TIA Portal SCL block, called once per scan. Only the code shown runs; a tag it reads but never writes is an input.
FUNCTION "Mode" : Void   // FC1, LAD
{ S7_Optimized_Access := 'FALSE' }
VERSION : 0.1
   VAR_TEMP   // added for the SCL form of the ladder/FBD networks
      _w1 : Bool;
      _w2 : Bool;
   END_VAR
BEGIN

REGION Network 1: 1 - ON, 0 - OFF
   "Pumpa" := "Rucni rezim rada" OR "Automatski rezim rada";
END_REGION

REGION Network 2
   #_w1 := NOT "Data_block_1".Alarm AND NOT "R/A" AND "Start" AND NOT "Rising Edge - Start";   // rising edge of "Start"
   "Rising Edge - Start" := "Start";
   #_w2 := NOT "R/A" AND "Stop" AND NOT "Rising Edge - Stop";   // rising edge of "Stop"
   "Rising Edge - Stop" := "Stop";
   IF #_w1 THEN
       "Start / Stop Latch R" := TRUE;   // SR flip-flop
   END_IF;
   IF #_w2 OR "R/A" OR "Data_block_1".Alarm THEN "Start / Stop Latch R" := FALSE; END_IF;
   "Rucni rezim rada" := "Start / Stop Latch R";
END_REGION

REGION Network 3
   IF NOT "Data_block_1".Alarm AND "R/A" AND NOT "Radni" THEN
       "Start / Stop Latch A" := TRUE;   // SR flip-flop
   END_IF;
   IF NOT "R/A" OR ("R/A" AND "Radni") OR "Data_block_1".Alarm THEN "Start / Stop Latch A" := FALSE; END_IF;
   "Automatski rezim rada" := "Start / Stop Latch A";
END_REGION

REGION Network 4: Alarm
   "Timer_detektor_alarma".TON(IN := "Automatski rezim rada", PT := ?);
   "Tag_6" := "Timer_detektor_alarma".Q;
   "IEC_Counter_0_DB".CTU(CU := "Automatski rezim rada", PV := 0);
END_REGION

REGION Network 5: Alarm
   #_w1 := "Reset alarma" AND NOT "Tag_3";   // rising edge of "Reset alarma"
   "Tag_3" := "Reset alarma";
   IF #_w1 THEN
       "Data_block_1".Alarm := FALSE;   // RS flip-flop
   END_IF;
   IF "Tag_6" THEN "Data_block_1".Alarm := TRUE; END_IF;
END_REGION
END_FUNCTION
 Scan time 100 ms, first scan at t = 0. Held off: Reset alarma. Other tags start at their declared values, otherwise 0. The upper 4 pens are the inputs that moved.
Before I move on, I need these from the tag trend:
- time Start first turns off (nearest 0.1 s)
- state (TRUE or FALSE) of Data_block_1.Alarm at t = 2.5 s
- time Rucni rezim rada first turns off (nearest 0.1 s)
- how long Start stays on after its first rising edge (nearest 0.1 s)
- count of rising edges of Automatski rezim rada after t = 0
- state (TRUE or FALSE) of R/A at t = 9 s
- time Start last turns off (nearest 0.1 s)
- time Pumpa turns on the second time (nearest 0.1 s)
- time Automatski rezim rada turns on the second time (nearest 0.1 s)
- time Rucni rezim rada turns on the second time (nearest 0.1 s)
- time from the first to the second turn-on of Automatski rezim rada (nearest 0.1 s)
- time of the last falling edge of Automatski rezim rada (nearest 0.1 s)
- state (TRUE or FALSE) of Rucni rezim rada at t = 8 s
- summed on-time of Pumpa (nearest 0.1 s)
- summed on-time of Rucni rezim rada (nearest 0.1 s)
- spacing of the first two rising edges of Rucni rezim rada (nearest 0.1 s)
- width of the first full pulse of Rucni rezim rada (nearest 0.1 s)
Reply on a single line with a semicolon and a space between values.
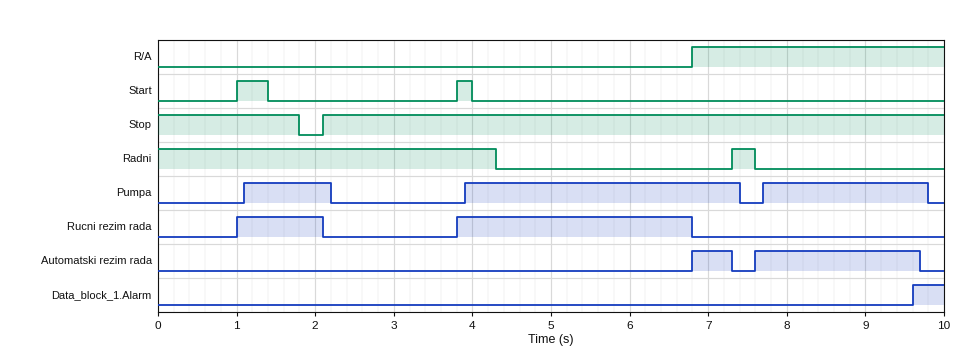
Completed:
1.4 s; FALSE; 2.1 s; 0.4 s; 2; TRUE; 4.0 s; 3.9 s; 7.6 s; 3.8 s; 0.8 s; 9.7 s; FALSE; 6.7 s; 4.1 s; 2.8 s; 1.1 s
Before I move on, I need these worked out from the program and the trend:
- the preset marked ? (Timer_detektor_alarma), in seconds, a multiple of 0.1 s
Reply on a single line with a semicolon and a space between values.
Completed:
2.0 s
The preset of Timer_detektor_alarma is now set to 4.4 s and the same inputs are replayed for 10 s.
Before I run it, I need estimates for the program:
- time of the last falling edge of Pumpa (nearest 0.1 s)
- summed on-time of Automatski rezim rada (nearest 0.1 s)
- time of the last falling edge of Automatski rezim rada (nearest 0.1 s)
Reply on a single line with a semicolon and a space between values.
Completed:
7.4 s; 2.9 s; 7.3 s
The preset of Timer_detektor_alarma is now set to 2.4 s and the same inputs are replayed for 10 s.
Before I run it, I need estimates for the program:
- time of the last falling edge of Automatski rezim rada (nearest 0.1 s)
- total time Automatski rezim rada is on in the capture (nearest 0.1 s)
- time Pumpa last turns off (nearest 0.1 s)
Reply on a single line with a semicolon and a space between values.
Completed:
7.3 s; 2.9 s; 7.4 s
